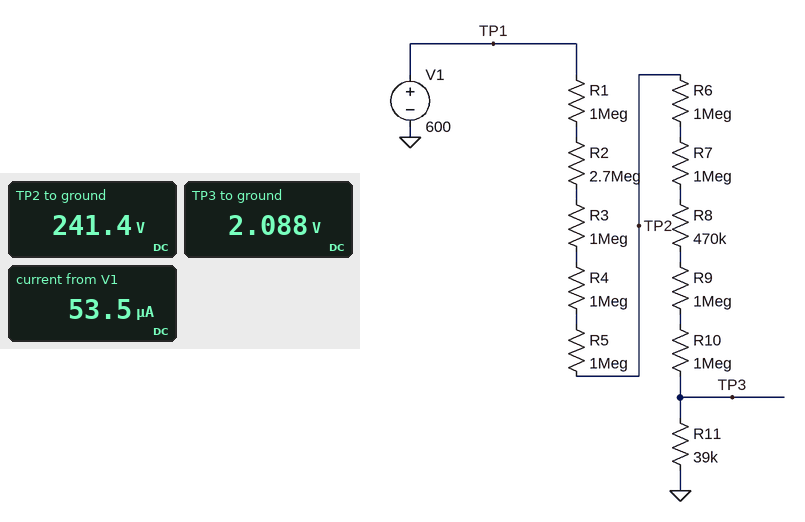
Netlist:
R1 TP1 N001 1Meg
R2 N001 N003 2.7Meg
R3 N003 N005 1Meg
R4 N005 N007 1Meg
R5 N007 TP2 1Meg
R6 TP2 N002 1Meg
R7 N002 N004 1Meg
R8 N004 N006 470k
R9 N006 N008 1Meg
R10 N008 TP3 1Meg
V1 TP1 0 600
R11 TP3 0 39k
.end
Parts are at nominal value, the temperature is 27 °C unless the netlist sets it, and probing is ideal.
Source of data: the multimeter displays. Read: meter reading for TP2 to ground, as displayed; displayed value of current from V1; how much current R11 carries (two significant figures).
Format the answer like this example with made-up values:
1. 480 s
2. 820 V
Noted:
1. 241.4 V
2. 53.5 µA
3. 54 µA
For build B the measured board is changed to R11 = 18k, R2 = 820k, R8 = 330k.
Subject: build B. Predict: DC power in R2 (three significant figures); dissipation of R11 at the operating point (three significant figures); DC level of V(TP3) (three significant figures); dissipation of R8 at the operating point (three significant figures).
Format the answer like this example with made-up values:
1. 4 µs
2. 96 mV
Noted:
1. 3.51 mW
2. 77.1 µW
3. 1.18 V
4. 1.41 mW
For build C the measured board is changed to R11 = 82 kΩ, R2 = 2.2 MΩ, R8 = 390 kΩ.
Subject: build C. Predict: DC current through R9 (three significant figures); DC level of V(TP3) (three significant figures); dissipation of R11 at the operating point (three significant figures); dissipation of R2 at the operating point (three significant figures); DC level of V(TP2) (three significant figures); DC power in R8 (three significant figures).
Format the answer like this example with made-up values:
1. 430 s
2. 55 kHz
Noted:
1. 56.2 µA
2. 4.61 V
3. 259 µW
4. 6.95 mW
5. 251 V
6. 1.23 mW
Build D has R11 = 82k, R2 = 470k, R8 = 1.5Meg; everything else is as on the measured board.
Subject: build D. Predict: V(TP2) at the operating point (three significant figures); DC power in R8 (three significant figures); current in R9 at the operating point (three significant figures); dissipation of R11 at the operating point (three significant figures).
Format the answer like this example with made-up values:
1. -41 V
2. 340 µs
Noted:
1. 333 V
2. 5.34 mW
3. 59.7 µA
4. 292 µW
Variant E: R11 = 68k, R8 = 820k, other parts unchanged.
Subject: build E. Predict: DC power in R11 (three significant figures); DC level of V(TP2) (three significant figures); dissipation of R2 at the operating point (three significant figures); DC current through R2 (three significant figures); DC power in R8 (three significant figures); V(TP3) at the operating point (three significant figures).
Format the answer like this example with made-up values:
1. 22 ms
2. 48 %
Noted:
1. 182 µW
2. 253 V
3. 7.24 mW
4. 51.8 µA
5. 2.20 mW
6. 3.52 V
